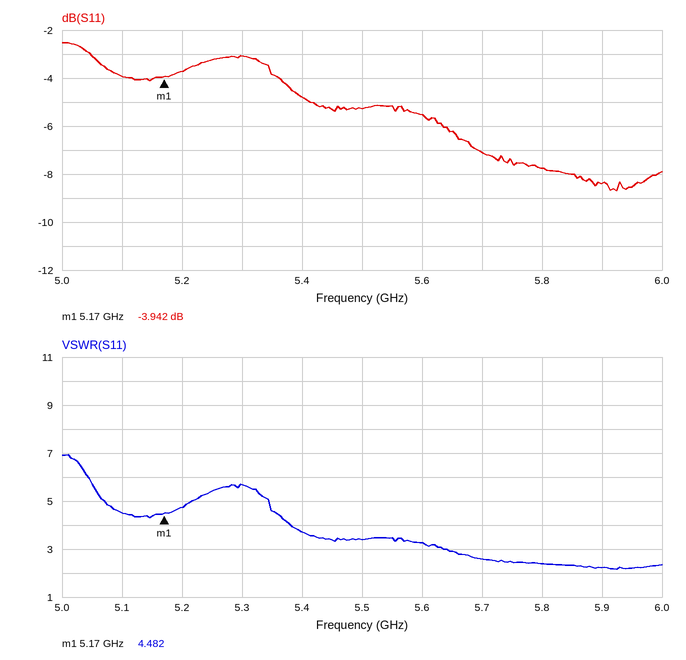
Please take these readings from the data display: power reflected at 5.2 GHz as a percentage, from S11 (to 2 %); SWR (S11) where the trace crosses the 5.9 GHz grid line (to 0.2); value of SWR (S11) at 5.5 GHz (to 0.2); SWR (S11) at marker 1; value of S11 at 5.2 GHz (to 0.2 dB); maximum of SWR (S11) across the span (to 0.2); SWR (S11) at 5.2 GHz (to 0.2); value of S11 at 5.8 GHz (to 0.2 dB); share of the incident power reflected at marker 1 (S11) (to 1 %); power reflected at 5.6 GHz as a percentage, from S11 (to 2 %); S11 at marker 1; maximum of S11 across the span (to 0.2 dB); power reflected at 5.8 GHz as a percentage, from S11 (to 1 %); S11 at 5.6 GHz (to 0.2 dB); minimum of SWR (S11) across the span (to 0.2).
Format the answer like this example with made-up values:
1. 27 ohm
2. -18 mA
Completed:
1. 42 %
2. 2.2
3. 3.4
4. 4.482
5. -3.8 dB
6. 7.0
7. 4.8
8. -7.8 dB
9. 40 %
10. 28 %
11. -3.942 dB
12. -2.6 dB
13. 17 %
14. -5.6 dB
15. 2.2
